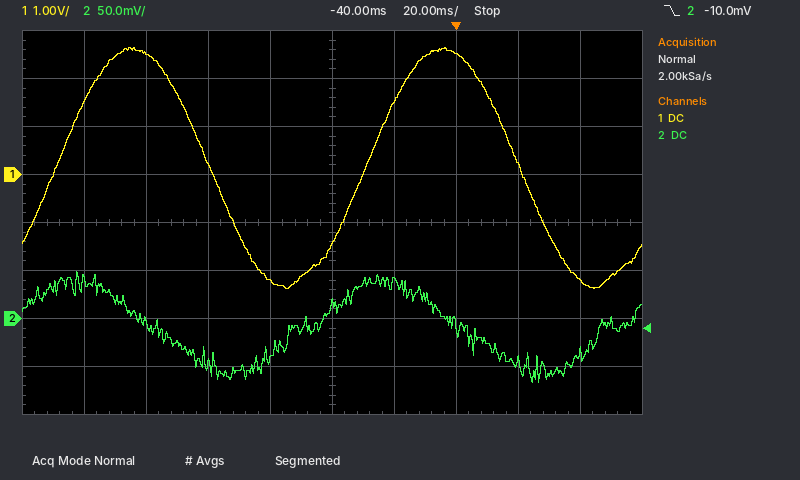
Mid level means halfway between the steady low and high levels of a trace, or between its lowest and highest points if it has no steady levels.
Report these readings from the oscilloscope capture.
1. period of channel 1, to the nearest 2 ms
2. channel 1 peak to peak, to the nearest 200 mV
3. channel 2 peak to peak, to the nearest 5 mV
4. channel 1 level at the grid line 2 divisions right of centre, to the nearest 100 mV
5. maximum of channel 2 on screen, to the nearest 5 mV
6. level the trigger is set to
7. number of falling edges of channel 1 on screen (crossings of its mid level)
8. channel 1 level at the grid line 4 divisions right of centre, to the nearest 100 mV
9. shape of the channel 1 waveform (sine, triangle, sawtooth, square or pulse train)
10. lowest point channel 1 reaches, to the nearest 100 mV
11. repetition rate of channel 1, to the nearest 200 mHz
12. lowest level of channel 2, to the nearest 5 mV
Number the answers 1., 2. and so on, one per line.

1. 100 ms
2. 5.0 V
3. 115 mV
4. 2.5 V
5. 50 mV
6. -10.0 mV
7. 2
8. -2.2 V
9. sine
10. -2.4 V
11. 10.0 Hz
12. -65 mV
